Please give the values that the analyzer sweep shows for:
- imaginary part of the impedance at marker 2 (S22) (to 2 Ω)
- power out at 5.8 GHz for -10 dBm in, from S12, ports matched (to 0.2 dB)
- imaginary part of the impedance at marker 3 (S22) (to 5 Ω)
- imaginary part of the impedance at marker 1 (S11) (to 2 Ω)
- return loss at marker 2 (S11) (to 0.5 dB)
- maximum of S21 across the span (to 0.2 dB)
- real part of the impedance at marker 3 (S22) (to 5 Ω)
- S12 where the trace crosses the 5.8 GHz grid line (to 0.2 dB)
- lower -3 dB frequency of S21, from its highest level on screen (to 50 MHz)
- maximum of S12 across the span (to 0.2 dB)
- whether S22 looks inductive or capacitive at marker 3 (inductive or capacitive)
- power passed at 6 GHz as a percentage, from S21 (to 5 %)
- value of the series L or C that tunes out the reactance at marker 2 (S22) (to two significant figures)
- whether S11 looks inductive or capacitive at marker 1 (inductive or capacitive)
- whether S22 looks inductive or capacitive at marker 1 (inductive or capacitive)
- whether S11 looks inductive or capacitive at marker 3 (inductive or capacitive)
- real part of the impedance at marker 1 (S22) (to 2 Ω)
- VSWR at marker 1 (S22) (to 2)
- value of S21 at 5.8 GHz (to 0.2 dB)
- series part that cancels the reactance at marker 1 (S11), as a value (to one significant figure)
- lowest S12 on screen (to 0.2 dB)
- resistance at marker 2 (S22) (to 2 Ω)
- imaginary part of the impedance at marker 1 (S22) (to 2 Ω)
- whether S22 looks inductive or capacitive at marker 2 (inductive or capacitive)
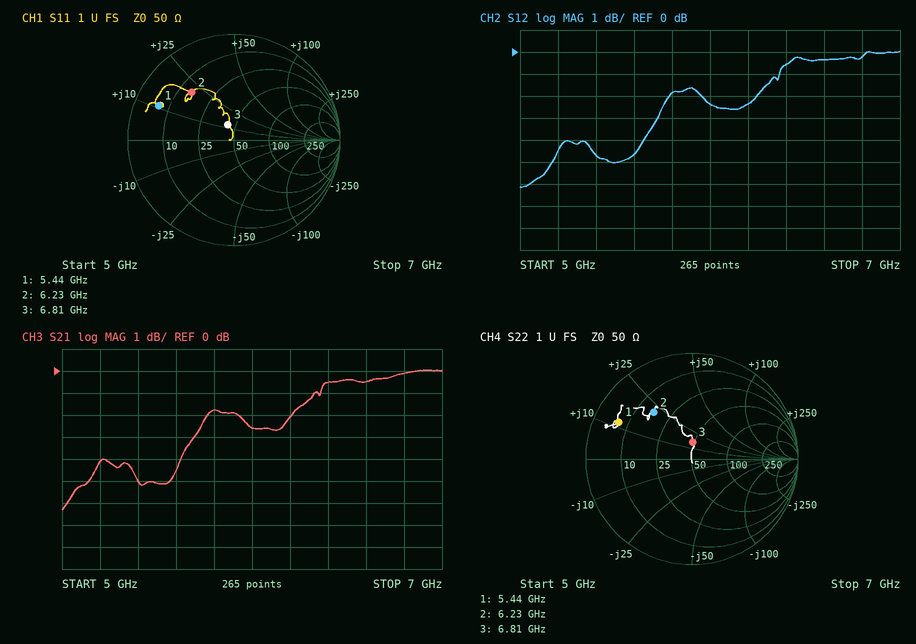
+22 Ω
-11.8 dBm
+15 Ω
+10 Ω
4.5 dB
0.0 dB
50 Ω
-1.8 dB
5.70 GHz
0.0 dB
inductive
55 %
1.2 pF
inductive
inductive
inductive
6 Ω
8
-1.8 dB
3 pF
-6.2 dB
16 Ω
+12 Ω
inductive
